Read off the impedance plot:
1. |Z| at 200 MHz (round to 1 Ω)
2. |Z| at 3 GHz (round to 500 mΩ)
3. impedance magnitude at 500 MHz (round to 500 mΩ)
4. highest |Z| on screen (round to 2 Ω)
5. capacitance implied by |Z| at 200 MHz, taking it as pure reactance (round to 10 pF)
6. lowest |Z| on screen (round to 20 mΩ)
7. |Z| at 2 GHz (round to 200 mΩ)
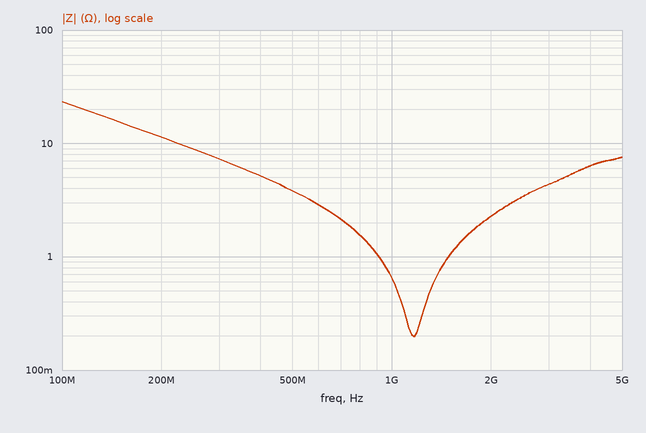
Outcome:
11 Ω
4.5 Ω
4.0 Ω
24 Ω
70 pF
200 mΩ
2.2 Ω
